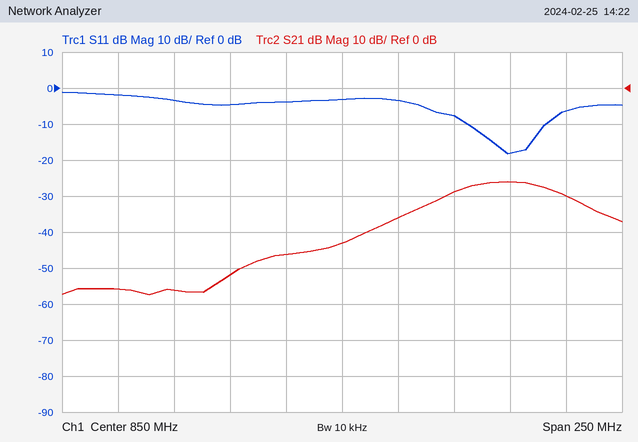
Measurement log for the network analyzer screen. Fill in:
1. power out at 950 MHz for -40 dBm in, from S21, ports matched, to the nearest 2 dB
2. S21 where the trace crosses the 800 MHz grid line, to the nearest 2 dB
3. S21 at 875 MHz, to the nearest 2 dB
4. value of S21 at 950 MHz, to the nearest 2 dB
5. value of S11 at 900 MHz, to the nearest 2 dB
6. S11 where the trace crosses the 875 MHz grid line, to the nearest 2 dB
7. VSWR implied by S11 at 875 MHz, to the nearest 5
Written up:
-70 dBm
-52 dB
-36 dB
-30 dB
-8 dB
-4 dB
5
